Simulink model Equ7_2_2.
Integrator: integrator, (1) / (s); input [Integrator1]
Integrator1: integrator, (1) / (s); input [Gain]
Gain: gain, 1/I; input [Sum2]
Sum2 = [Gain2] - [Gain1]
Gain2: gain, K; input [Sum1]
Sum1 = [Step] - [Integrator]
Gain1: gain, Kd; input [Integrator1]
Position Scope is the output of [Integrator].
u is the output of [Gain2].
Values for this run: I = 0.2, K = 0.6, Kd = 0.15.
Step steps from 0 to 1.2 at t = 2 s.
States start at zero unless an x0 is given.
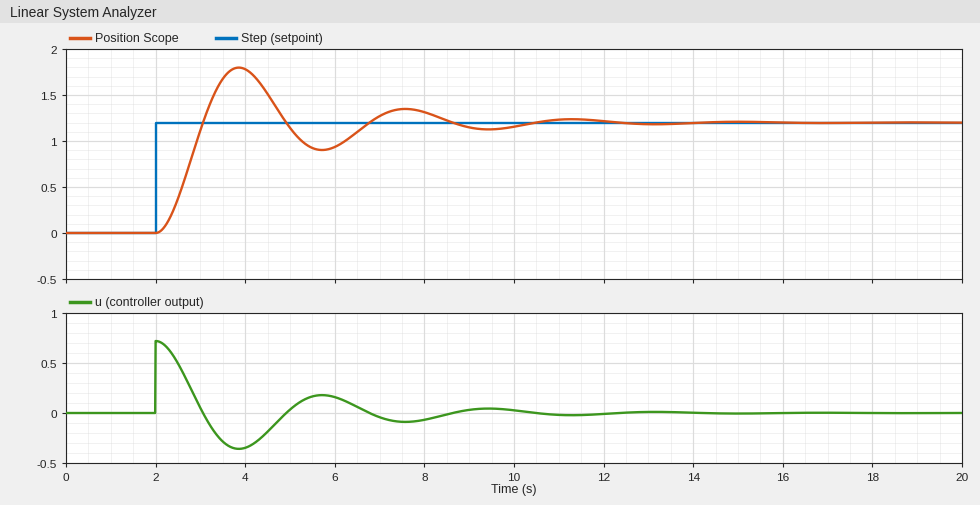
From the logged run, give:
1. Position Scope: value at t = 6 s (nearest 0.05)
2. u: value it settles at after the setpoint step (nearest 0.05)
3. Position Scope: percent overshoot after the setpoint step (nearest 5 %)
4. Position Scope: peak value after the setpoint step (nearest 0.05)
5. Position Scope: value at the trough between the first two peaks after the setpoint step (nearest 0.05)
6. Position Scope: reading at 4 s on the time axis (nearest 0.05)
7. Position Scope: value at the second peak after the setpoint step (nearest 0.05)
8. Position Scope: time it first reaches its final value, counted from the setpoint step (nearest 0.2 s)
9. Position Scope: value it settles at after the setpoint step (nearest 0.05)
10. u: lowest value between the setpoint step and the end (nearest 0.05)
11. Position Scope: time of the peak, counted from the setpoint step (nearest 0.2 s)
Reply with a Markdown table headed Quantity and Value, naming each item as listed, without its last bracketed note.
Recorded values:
| Quantity | Value |
|---|---|
| Position Scope: value at t = 6 s | 0.95 |
| u: value it settles at after the setpoint step | 0.00 |
| Position Scope: percent overshoot after the setpoint step | 50 % |
| Position Scope: peak value after the setpoint step | 1.80 |
| Position Scope: value at the trough between the first two peaks after the setpoint step | 0.90 |
| Position Scope: reading at 4 s on the time axis | 1.80 |
| Position Scope: value at the second peak after the setpoint step | 1.35 |
| Position Scope: time it first reaches its final value, counted from the setpoint step | 1.0 s |
| Position Scope: value it settles at after the setpoint step | 1.20 |
| u: lowest value between the setpoint step and the end | -0.35 |
| Position Scope: time of the peak, counted from the setpoint step | 1.8 s |
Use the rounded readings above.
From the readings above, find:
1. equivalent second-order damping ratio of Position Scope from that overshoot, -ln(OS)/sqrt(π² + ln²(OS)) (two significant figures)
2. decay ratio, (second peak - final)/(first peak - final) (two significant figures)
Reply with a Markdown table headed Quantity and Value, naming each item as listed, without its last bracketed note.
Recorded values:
| Quantity | Value |
|---|---|
| equivalent second-order damping ratio of Position Scope from that overshoot, -ln(OS)/sqrt(π² + ln²(OS)) | 0.22 |
| decay ratio, (second peak - final)/(first peak - final) | 0.25 |
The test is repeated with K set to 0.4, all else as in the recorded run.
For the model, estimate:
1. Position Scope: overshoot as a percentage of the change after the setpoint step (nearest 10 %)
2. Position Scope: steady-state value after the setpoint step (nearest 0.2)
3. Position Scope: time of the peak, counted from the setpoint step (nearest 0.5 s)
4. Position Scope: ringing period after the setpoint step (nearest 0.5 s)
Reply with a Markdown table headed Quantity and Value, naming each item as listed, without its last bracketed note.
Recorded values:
| Quantity | Value |
|---|---|
| Position Scope: overshoot as a percentage of the change after the setpoint step | 40 % |
| Position Scope: steady-state value after the setpoint step | 1.2 |
| Position Scope: time of the peak, counted from the setpoint step | 2.5 s |
| Position Scope: ringing period after the setpoint step | 4.5 s |
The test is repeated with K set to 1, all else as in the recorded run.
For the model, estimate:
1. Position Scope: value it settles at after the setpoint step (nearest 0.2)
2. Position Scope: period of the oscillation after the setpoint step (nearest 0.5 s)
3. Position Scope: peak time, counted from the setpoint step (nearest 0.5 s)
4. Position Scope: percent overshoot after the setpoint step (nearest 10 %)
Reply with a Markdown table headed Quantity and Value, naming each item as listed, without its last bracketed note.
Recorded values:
| Quantity | Value |
|---|---|
| Position Scope: value it settles at after the setpoint step | 1.2 |
| Position Scope: period of the oscillation after the setpoint step | 3.0 s |
| Position Scope: peak time, counted from the setpoint step | 1.5 s |
| Position Scope: percent overshoot after the setpoint step | 60 % |
